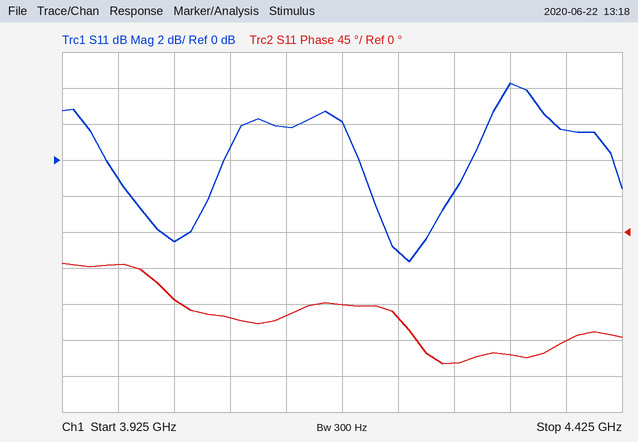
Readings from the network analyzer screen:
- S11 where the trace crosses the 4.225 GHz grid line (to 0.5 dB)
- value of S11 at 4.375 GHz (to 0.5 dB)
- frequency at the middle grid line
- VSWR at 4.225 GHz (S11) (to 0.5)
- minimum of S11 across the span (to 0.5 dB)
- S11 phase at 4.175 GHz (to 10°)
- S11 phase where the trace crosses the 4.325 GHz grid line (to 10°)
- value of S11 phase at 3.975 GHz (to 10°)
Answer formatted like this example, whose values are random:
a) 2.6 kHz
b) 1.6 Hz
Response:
a) -5.0 dB
b) 1.5 dB
c) 4.175 GHz
d) 3.5
e) -5.5 dB
f) -90°
g) -150°
h) -40°
